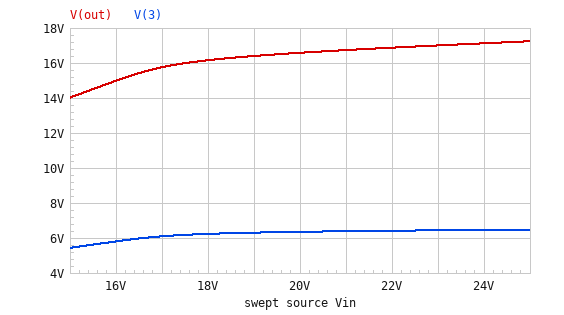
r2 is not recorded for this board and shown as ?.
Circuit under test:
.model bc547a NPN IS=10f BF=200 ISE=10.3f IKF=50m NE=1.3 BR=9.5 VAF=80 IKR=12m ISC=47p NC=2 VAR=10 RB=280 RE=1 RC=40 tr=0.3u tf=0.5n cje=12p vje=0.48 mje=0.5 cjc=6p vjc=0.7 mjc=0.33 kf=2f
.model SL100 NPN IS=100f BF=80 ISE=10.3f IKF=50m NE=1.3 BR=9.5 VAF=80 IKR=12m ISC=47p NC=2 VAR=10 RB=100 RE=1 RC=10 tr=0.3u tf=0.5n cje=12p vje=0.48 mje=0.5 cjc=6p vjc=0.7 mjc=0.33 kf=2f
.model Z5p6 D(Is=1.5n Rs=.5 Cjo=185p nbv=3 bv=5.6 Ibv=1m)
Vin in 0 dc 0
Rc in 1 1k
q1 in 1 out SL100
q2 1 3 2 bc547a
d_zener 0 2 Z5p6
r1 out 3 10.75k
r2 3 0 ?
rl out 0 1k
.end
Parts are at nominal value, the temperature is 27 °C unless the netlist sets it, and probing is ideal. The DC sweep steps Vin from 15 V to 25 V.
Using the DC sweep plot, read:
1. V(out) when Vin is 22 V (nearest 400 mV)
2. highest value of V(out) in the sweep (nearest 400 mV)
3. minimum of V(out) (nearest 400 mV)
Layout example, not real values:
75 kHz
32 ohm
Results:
16.8 V
17.2 V
14.0 V
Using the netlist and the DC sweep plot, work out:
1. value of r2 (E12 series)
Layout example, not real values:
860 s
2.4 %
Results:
6.8 kΩ
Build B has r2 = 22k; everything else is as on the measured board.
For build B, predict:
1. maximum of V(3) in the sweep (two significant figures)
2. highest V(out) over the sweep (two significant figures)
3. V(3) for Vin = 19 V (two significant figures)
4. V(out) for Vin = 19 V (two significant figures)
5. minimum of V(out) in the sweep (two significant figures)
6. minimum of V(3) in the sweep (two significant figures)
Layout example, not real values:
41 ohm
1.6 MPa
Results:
6.6 V
11 V
6.5 V
10 V
9.9 V
6.4 V
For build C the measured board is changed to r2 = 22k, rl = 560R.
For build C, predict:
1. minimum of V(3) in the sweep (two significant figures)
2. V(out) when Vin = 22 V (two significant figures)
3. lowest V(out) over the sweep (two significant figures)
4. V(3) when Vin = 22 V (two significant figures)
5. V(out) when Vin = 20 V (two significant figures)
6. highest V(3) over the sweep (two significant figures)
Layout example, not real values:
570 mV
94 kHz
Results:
6.4 V
11 V
9.9 V
6.5 V
10 V
6.6 V
